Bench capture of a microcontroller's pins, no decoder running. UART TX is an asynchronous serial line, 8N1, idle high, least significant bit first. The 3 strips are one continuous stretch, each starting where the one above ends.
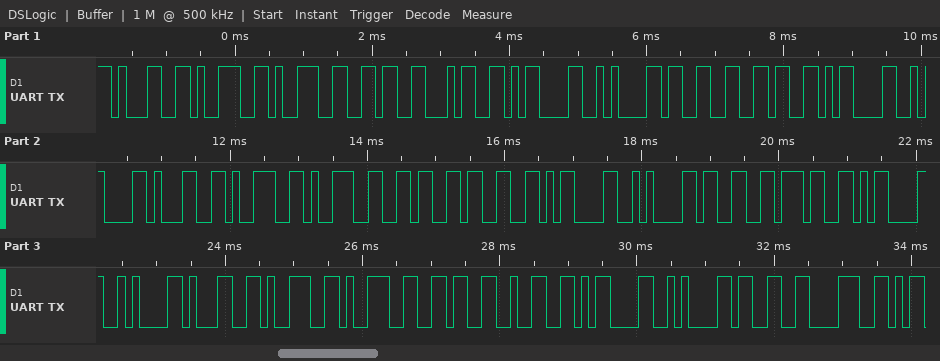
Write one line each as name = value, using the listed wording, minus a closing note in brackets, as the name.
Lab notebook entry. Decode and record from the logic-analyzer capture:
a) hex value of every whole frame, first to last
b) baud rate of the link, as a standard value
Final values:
hex value of every whole frame, first to last = 31 39 39 36 34 0D 0A 33 36 0D 0A 31 39 39 36 33 0D 0A 33 37 0D 0A 31 39 39 36 32 0D 0A 33 38
baud rate of the link, as a standard value = 9600 baud
